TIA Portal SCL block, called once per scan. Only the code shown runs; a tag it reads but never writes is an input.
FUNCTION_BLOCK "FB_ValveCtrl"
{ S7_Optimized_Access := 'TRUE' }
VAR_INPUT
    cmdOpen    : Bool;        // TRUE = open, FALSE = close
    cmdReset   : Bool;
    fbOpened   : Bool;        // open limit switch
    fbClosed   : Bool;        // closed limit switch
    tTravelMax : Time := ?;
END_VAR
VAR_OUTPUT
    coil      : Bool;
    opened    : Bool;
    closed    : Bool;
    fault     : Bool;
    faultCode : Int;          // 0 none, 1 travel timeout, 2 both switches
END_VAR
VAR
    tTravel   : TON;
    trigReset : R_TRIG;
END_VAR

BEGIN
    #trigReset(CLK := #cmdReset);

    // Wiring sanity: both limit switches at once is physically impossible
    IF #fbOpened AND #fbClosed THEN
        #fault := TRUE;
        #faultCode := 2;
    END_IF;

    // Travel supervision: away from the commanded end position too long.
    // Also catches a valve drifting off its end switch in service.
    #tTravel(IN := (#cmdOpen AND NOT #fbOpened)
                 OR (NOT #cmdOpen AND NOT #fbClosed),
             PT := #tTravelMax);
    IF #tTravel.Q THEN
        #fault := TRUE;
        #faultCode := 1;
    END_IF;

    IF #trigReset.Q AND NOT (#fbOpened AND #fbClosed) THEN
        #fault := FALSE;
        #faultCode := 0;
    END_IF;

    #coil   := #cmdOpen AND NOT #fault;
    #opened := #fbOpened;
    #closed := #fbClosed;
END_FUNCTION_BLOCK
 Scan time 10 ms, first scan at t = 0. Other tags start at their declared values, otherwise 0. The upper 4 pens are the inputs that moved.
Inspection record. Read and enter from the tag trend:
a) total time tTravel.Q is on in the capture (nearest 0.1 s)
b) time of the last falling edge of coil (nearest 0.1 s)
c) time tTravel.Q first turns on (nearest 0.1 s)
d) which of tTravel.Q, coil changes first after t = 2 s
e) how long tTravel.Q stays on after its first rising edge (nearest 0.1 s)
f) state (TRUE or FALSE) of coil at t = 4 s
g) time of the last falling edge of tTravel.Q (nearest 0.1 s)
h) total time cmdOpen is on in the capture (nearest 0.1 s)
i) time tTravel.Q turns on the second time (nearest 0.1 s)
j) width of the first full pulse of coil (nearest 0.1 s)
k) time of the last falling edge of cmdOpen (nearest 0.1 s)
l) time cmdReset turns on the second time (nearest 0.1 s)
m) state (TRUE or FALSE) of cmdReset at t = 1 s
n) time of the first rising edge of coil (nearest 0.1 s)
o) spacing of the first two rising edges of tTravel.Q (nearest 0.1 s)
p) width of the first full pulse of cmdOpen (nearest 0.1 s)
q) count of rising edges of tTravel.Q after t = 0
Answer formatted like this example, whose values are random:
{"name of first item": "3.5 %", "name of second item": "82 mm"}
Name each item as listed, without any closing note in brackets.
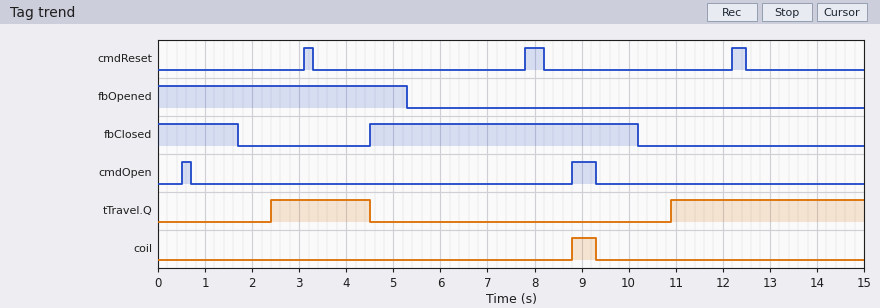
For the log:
{"total time tTravel.Q is on in the capture": "6.2 s", "time of the last falling edge of coil": "9.3 s", "time tTravel.Q first turns on": "2.4 s", "which of tTravel.Q, coil changes first after t = 2 s": "tTravel.Q", "how long tTravel.Q stays on after its first rising edge": "2.1 s", "state (TRUE or FALSE) of coil at t = 4 s": "FALSE", "time of the last falling edge of tTravel.Q": "4.5 s", "total time cmdOpen is on in the capture": "0.7 s", "time tTravel.Q turns on the second time": "10.9 s", "width of the first full pulse of coil": "0.5 s", "time of the last falling edge of cmdOpen": "9.3 s", "time cmdReset turns on the second time": "7.8 s", "state (TRUE or FALSE) of cmdReset at t = 1 s": "FALSE", "time of the first rising edge of coil": "8.8 s", "spacing of the first two rising edges of tTravel.Q": "8.5 s", "width of the first full pulse of cmdOpen": "0.2 s", "count of rising edges of tTravel.Q after t = 0": "2"}
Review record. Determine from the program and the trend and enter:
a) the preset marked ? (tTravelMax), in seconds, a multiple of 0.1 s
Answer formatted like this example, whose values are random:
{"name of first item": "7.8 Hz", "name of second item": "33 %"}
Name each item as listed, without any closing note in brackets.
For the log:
{"the preset marked ? (tTravelMax), in seconds, a multiple of 0.1 s": "0.7 s"}
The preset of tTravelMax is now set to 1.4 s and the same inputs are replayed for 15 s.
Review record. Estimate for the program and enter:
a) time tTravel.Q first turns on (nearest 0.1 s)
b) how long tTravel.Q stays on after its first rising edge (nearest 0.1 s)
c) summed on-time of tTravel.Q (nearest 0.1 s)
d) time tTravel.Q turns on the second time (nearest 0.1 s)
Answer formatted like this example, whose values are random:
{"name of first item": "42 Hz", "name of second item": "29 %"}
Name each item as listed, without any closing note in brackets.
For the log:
{"time tTravel.Q first turns on": "3.1 s", "how long tTravel.Q stays on after its first rising edge": "1.4 s", "summed on-time of tTravel.Q": "4.8 s", "time tTravel.Q turns on the second time": "11.6 s"}
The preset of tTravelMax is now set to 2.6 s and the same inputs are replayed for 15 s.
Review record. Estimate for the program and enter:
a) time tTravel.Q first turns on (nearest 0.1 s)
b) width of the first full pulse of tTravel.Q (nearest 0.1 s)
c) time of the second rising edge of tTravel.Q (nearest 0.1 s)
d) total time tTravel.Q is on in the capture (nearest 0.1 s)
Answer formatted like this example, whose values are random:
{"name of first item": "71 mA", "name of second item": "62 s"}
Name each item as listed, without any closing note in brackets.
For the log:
{"time tTravel.Q first turns on": "4.3 s", "width of the first full pulse of tTravel.Q": "0.2 s", "time of the second rising edge of tTravel.Q": "12.8 s", "total time tTravel.Q is on in the capture": "2.4 s"}
